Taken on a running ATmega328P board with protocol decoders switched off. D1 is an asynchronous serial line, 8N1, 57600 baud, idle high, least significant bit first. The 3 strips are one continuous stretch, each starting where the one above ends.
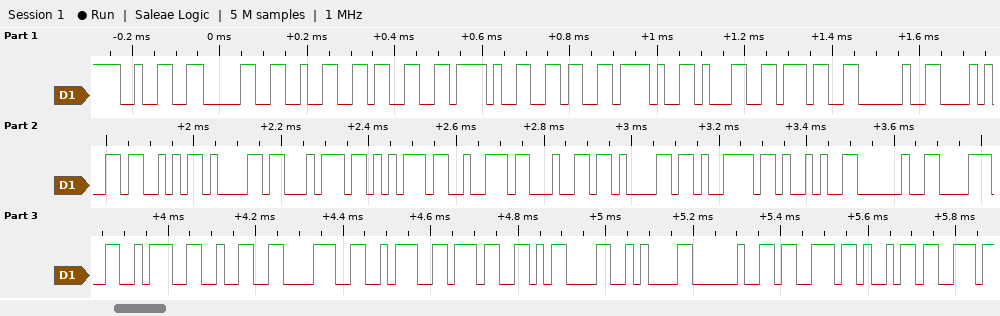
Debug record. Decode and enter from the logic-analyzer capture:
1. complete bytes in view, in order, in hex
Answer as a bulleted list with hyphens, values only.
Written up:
- 32 30 32 33 2F 36 2F 31 37 20 28 53 61 74 75 72 64 61 79 29 20 38 3A 32 38 3A 37 0D 0A 20 73 69
